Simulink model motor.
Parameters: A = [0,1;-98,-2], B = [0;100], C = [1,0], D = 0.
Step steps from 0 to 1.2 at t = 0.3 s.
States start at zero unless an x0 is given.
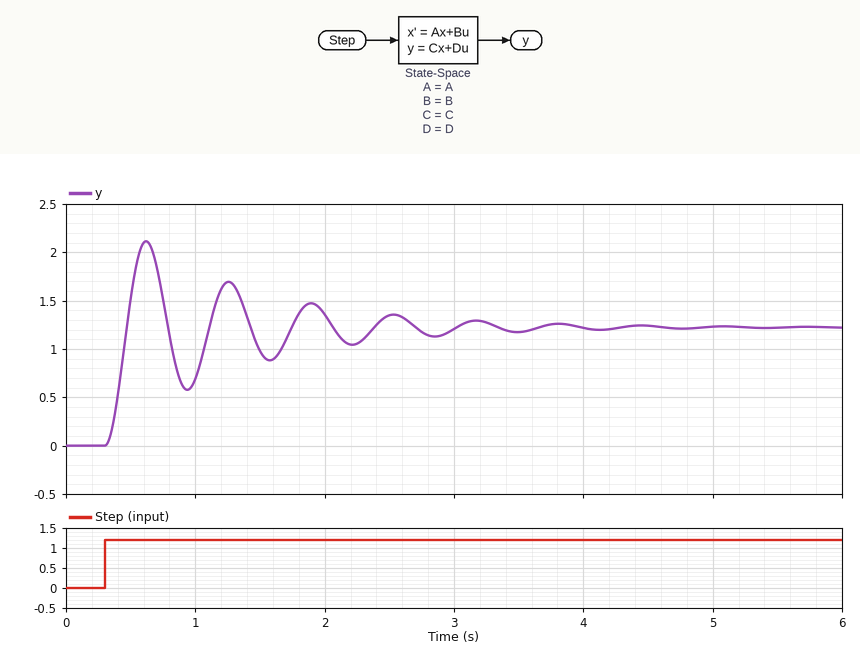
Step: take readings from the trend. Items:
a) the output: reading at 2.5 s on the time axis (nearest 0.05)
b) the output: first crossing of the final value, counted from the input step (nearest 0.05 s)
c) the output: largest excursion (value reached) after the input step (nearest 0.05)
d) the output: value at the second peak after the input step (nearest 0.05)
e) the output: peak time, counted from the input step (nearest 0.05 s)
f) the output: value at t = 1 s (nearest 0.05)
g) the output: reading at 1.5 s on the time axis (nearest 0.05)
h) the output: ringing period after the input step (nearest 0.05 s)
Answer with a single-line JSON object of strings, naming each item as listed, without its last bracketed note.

{"the output: reading at 2.5 s on the time axis": "1.35", "the output: first crossing of the final value, counted from the input step": "0.15 s", "the output: largest excursion (value reached) after the input step": "2.10", "the output: value at the second peak after the input step": "1.70", "the output: peak time, counted from the input step": "0.30 s", "the output: value at t = 1 s": "0.70", "the output: reading at 1.5 s on the time axis": "1.00", "the output: ringing period after the input step": "0.65 s"}
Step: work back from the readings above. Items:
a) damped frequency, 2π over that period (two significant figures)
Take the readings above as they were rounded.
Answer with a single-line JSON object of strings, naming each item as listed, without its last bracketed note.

{"damped frequency, 2π over that period": "9.7 rad/s"}
